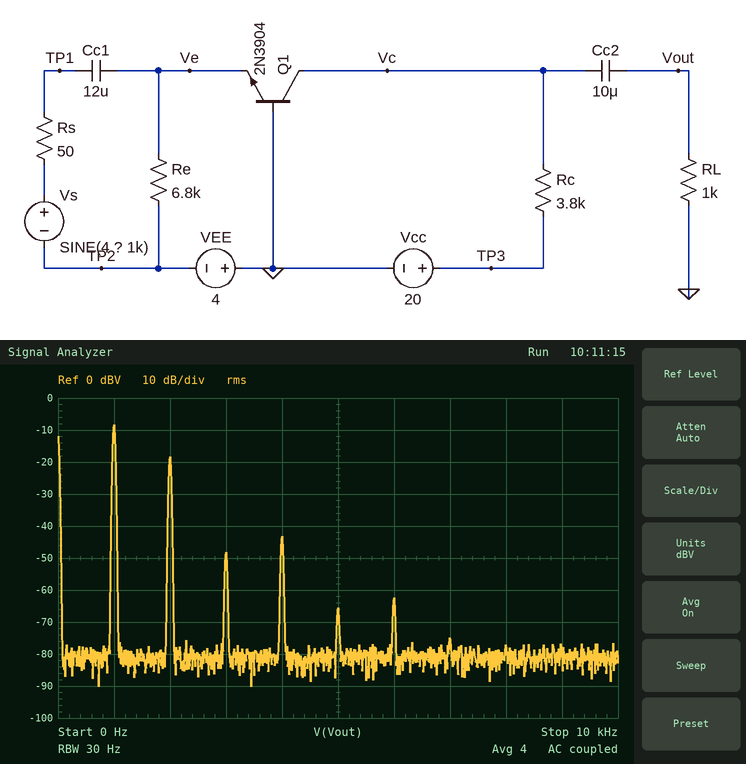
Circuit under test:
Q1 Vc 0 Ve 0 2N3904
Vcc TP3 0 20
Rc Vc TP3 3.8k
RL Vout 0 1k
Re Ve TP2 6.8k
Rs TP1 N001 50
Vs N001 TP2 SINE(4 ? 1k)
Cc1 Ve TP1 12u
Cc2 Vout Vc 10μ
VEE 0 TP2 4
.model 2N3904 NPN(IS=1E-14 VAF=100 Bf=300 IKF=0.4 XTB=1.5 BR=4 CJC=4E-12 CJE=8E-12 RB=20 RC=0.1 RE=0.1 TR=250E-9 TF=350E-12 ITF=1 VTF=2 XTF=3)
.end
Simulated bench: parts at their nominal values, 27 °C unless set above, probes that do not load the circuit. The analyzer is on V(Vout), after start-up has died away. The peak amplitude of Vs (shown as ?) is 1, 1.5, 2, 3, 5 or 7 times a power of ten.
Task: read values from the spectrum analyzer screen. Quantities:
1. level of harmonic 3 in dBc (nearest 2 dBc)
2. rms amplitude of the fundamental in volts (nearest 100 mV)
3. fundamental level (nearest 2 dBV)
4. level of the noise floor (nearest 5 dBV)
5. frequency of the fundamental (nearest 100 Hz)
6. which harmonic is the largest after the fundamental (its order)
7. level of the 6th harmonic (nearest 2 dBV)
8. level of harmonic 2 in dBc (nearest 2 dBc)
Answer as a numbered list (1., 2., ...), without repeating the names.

1. -40 dBc
2. 400 mV
3. -8 dBV
4. -80 dBV
5. 1.0 kHz
6. 2
7. -62 dBV
8. -10 dBc
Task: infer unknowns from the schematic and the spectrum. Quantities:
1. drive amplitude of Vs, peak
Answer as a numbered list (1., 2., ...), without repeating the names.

1. 100 mV
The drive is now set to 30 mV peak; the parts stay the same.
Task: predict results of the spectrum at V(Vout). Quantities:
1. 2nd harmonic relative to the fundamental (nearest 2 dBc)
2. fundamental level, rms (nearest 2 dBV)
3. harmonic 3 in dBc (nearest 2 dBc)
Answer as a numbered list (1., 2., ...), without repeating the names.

1. -22 dBc
2. -16 dBV
3. -50 dBc
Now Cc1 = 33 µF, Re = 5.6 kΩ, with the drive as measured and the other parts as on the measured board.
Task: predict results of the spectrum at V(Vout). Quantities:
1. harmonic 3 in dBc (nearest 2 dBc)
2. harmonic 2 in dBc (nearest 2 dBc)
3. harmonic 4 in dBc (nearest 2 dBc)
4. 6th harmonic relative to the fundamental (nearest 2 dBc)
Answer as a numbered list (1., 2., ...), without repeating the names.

1. -42 dBc
2. -12 dBc
3. -38 dBc
4. -60 dBc
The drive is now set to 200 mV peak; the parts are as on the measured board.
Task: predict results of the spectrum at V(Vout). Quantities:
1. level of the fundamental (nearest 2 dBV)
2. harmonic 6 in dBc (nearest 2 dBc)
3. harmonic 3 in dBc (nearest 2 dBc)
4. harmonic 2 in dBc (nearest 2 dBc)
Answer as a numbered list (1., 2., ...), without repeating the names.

1. -6 dBV
2. -48 dBc
3. -16 dBc
4. -6 dBc
